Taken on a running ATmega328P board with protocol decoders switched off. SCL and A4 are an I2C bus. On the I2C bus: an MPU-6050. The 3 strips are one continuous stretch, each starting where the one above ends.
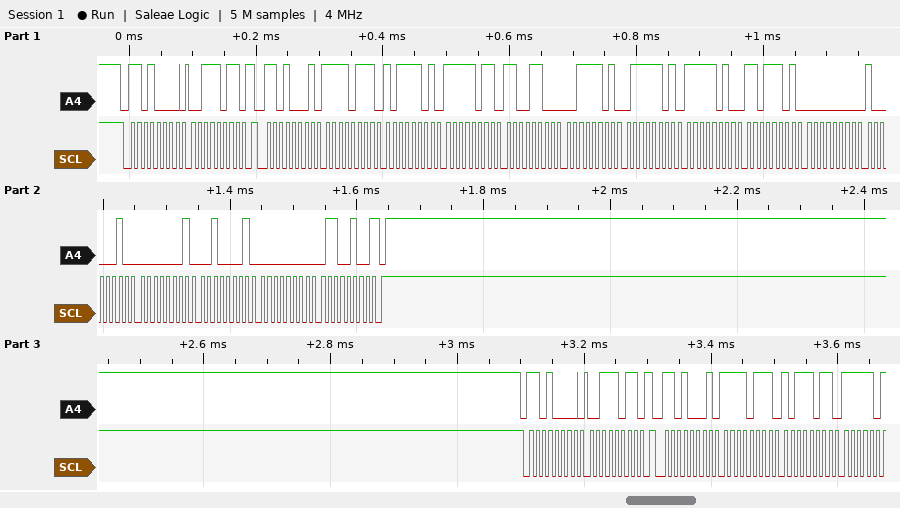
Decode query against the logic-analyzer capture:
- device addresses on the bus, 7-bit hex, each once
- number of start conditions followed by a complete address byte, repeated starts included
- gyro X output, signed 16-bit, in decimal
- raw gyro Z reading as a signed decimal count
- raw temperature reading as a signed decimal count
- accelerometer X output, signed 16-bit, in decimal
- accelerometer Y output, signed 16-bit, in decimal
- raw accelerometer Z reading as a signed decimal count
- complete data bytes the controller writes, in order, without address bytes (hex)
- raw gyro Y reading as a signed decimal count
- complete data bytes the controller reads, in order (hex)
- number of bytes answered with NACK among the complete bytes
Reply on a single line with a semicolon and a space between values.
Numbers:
0x68; 4; 130; 100; -1315; -2115; -1076; 15741; 3B 3B; 289; F7 BD FB CC 3D 7D FA DD 00 82 01 21 00 64 F7 BB; 1
